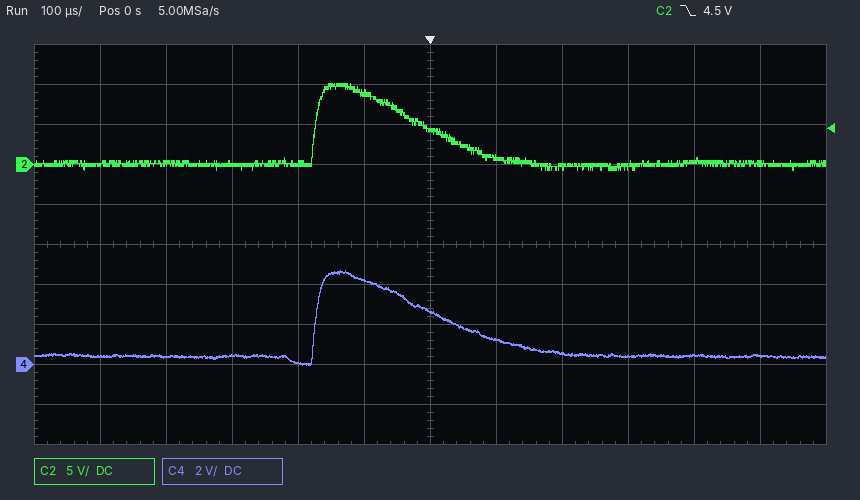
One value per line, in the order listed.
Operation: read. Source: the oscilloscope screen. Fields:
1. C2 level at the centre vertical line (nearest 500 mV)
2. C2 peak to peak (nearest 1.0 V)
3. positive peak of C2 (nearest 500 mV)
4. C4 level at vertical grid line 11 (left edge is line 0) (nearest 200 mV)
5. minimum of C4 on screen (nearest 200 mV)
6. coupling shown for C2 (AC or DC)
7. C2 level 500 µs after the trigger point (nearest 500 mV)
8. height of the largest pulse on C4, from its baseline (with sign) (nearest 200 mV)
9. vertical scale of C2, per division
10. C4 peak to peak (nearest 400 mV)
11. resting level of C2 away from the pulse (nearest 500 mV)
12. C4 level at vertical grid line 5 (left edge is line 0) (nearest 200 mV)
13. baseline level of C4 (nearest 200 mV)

4.5 V
11.0 V
10.0 V
400 mV
0.0 V
DC
0.0 V
+4.2 V
5 V
4.8 V
0.0 V
4.2 V
400 mV
